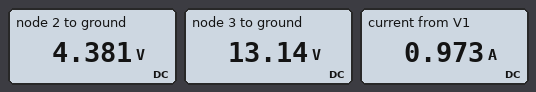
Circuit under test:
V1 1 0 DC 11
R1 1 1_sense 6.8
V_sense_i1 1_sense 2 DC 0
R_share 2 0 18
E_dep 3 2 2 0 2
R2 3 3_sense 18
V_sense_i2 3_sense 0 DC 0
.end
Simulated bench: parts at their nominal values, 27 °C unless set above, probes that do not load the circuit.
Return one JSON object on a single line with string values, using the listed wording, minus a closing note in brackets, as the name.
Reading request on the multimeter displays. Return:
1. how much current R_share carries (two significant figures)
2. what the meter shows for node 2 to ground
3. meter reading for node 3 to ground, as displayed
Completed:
{"how much current R_share carries": "240 mA", "what the meter shows for node 2 to ground": "4.381 V", "meter reading for node 3 to ground, as displayed": "13.14 V"}
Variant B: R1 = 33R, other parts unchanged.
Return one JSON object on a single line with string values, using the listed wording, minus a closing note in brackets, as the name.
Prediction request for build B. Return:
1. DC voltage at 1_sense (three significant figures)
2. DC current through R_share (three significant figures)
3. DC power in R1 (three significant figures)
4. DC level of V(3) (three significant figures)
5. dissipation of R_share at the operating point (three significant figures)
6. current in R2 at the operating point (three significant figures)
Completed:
{"DC voltage at 1_sense": "1.32 V", "DC current through R_share": "73.3 mA", "DC power in R1": "2.84 W", "DC level of V(3)": "3.96 V", "dissipation of R_share at the operating point": "96.8 mW", "current in R2 at the operating point": "220 mA"}
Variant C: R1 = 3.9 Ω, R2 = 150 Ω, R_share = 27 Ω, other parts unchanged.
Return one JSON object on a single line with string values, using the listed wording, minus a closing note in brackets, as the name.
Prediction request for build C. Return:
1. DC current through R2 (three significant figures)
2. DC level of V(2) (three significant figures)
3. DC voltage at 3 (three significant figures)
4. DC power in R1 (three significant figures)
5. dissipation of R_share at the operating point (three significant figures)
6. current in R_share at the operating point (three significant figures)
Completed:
{"DC current through R2": "180 mA", "DC level of V(2)": "9.00 V", "DC voltage at 3": "27.0 V", "DC power in R1": "1.03 W", "dissipation of R_share at the operating point": "3.00 W", "current in R_share at the operating point": "333 mA"}
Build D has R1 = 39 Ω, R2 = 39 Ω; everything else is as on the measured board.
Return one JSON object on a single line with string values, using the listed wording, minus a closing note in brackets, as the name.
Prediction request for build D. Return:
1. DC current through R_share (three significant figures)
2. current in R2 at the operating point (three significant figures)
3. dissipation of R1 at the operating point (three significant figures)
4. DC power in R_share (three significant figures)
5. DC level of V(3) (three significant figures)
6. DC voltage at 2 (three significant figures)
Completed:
{"DC current through R_share": "99.1 mA", "current in R2 at the operating point": "137 mA", "dissipation of R1 at the operating point": "2.18 W", "DC power in R_share": "177 mW", "DC level of V(3)": "5.35 V", "DC voltage at 2": "1.78 V"}
